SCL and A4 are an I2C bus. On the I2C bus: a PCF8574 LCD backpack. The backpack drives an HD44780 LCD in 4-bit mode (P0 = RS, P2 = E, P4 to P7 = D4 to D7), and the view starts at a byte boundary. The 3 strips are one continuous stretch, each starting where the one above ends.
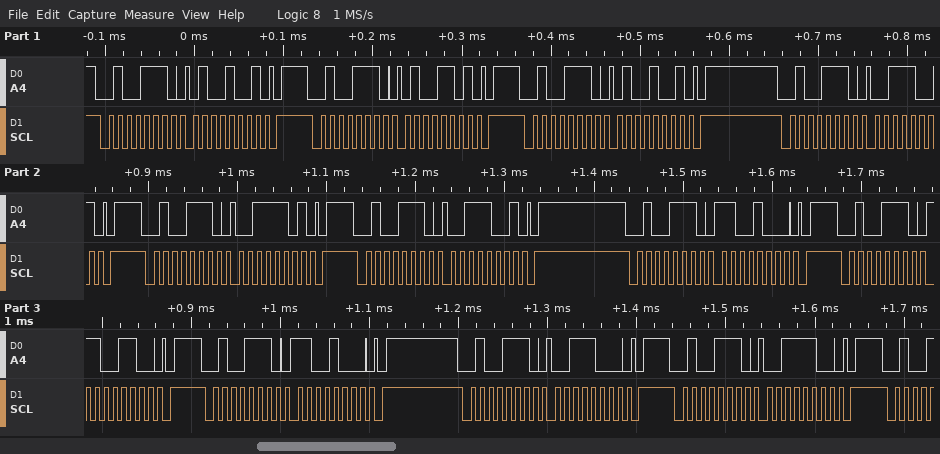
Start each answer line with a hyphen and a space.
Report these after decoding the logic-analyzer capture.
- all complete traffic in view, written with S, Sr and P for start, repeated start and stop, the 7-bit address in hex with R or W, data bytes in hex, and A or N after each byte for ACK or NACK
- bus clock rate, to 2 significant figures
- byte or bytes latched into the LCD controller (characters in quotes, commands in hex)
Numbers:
- S 27W A 49 A P S 27W A 4D A P S 27W A 49 A P S 27W A 39 A P S 27W A 3D A P S 27W A 39 A P S 27W A C8 A P S 27W A CC A P S 27W A C8 A P S 27W A 38 A P S 27W A 3C A P
- 100 kHz
- 'C'
